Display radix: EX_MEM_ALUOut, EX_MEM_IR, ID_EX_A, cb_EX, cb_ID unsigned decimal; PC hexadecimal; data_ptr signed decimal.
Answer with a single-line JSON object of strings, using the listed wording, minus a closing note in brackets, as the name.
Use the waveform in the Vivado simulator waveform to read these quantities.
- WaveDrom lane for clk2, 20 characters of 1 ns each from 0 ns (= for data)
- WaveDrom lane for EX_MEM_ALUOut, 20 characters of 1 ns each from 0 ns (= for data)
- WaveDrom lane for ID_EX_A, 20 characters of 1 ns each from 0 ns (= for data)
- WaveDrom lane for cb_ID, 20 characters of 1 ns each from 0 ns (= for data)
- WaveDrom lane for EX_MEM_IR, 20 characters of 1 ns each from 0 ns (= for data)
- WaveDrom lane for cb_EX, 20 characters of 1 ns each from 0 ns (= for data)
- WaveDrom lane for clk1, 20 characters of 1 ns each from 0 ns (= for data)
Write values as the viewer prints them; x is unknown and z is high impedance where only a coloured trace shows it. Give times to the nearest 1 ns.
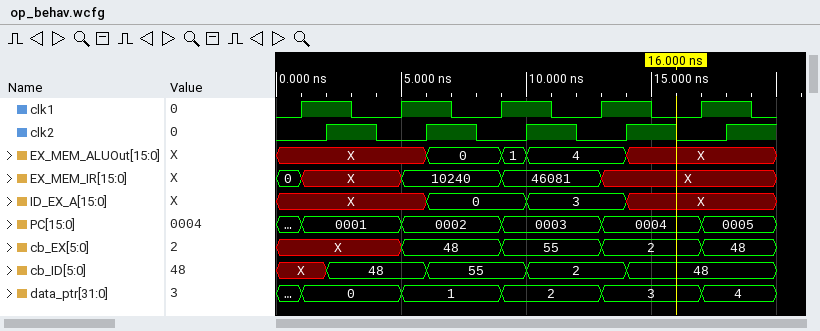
{"WaveDrom lane for clk2, 20 characters of 1 ns each from 0 ns": "{name: 'clk2', wave: '0.1.0.1.0.1.0.1.0.1.'}", "WaveDrom lane for EX_MEM_ALUOut, 20 characters of 1 ns each from 0 ns": "{name: 'EX_MEM_ALUOut', wave: 'x.....=..==...x.....', data: '0 1 4'}", "WaveDrom lane for ID_EX_A, 20 characters of 1 ns each from 0 ns": "{name: 'ID_EX_A', wave: 'x.....=...=...x.....', data: '0 3'}", "WaveDrom lane for cb_ID, 20 characters of 1 ns each from 0 ns": "{name: 'cb_ID', wave: 'x.=...=...=...=.....', data: '48 55 2 48'}", "WaveDrom lane for EX_MEM_IR, 20 characters of 1 ns each from 0 ns": "{name: 'EX_MEM_IR', wave: '=x...=...=...x......', data: '0 10240 46081'}", "WaveDrom lane for cb_EX, 20 characters of 1 ns each from 0 ns": "{name: 'cb_EX', wave: 'x....=...=...=...=..', data: '48 55 2 48'}", "WaveDrom lane for clk1, 20 characters of 1 ns each from 0 ns": "{name: 'clk1', wave: '01.0.1.0.1.0.1.0.1.0'}"}
